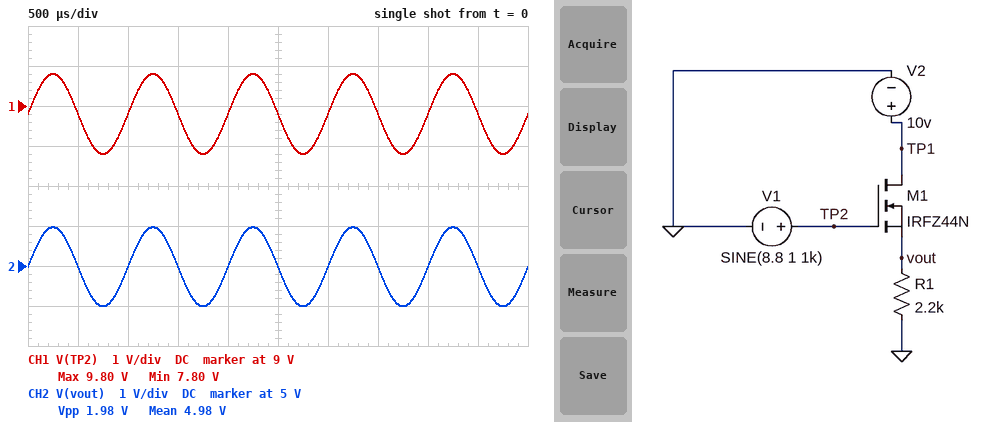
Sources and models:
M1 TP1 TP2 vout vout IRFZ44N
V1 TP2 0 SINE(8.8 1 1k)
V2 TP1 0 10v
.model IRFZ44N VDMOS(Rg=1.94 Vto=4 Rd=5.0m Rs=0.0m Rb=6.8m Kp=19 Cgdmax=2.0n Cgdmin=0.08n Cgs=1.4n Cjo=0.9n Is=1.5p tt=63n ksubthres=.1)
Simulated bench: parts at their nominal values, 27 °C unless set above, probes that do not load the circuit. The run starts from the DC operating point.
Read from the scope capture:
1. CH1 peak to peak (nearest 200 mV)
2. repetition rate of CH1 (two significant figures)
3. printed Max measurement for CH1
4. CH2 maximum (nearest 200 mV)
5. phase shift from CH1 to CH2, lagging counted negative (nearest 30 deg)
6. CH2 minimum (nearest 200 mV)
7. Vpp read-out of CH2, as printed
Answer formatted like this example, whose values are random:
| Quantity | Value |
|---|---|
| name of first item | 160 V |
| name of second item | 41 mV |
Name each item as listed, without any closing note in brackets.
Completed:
| Quantity | Value |
|---|---|
| CH1 peak to peak | 2.0 V |
| repetition rate of CH1 | 1.0 kHz |
| printed Max measurement for CH1 | 9.80 V |
| CH2 maximum | 6.0 V |
| phase shift from CH1 to CH2, lagging counted negative | 0 deg |
| CH2 minimum | 4.0 V |
| Vpp read-out of CH2, as printed | 1.98 V |
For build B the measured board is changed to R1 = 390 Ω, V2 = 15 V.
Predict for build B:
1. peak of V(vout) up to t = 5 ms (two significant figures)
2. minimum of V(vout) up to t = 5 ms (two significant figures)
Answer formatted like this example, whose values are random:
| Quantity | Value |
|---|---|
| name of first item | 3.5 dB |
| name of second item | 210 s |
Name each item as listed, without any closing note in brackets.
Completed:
| Quantity | Value |
|---|---|
| peak of V(vout) up to t = 5 ms | 5.9 V |
| minimum of V(vout) up to t = 5 ms | 3.9 V |
